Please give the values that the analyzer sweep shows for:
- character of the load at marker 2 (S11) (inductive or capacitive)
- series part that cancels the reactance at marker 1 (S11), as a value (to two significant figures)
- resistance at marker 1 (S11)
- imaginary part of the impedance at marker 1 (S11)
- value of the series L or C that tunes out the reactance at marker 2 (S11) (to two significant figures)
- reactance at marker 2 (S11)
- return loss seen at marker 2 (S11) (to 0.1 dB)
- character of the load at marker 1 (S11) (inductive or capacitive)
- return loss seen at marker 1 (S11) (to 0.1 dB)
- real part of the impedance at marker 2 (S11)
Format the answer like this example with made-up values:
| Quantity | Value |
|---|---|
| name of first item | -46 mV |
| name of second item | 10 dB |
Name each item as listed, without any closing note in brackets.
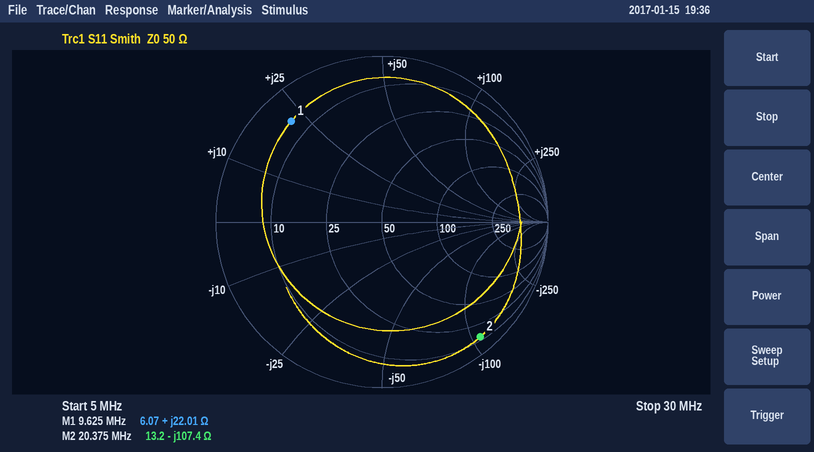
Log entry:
| Quantity | Value |
|---|---|
| character of the load at marker 2 (S11) | capacitive |
| series part that cancels the reactance at marker 1 (S11), as a value | 750 pF |
| resistance at marker 1 | 6.07 Ω |
| imaginary part of the impedance at marker 1 | +22.01 Ω |
| value of the series L or C that tunes out the reactance at marker 2 (S11) | 840 nH |
| reactance at marker 2 | -107.4 Ω |
| return loss seen at marker 2 (S11) | 0.8 dB |
| character of the load at marker 1 (S11) | inductive |
| return loss seen at marker 1 (S11) | 1.8 dB |
| real part of the impedance at marker 2 | 13.2 Ω |
